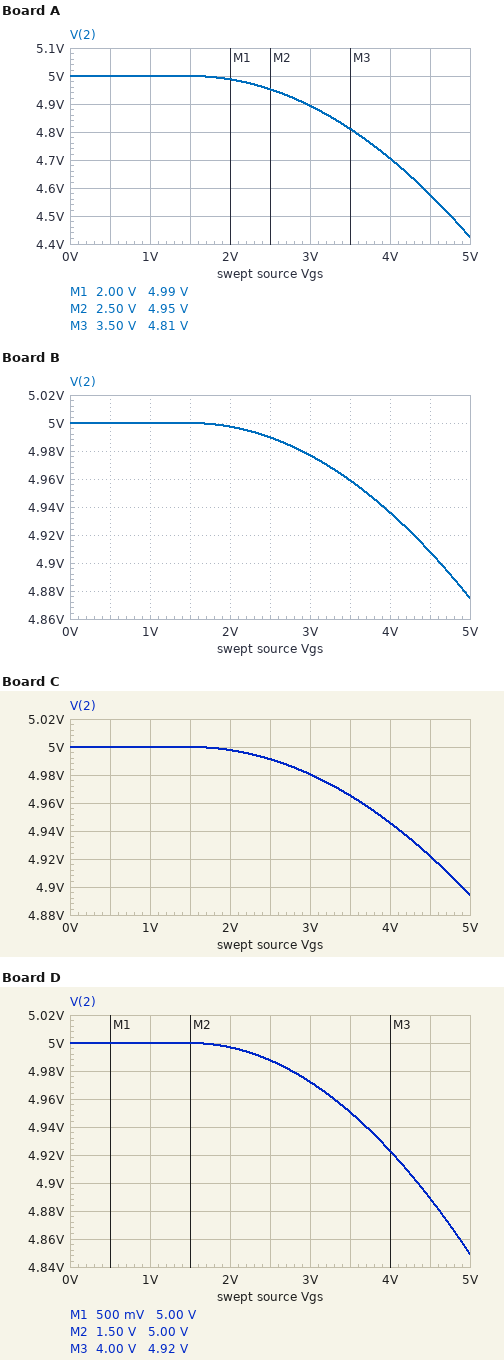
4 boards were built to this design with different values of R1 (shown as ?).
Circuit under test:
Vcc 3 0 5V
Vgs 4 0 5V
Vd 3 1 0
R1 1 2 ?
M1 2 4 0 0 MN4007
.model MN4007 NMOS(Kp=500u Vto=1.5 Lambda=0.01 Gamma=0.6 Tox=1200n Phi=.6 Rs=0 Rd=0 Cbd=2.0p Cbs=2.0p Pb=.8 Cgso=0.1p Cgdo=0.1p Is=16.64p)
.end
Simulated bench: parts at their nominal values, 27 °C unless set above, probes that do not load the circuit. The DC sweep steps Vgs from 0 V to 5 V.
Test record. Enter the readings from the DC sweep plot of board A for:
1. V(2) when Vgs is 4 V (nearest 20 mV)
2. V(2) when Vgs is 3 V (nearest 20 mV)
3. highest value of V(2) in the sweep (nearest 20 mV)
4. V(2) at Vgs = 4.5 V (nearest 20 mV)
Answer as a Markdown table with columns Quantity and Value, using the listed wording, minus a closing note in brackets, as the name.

| Quantity | Value |
|---|---|
| V(2) when Vgs is 4 V | 4.70 V |
| V(2) when Vgs is 3 V | 4.90 V |
| highest value of V(2) in the sweep | 5.00 V |
| V(2) at Vgs = 4.5 V | 4.58 V |
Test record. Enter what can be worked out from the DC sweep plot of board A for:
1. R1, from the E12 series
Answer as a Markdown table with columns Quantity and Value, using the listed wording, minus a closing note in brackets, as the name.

| Quantity | Value |
|---|---|
| R1, from the E12 series | 180 Ω |
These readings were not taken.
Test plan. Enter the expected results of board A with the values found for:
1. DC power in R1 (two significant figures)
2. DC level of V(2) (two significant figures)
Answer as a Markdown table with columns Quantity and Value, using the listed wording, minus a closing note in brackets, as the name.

| Quantity | Value |
|---|---|
| DC power in R1 | 1.8 mW |
| DC level of V(2) | 4.4 V |
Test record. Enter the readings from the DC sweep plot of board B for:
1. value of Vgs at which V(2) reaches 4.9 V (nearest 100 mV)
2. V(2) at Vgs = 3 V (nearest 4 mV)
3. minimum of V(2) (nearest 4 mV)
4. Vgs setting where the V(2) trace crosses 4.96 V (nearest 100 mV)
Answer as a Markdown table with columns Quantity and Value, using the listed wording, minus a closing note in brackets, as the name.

| Quantity | Value |
|---|---|
| value of Vgs at which V(2) reaches 4.9 V | 4.6 V |
| V(2) at Vgs = 3 V | 4.976 V |
| minimum of V(2) | 4.876 V |
| Vgs setting where the V(2) trace crosses 4.96 V | 3.5 V |
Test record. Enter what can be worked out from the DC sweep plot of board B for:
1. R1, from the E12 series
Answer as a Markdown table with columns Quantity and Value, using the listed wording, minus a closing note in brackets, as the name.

| Quantity | Value |
|---|---|
| R1, from the E12 series | 39 Ω |
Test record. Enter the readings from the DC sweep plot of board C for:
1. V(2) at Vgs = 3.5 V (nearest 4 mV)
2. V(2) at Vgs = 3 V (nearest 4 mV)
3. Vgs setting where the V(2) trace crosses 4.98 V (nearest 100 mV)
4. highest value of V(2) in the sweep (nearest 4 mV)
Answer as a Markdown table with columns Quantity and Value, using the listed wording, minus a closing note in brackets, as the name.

| Quantity | Value |
|---|---|
| V(2) at Vgs = 3.5 V | 4.964 V |
| V(2) at Vgs = 3 V | 4.980 V |
| Vgs setting where the V(2) trace crosses 4.98 V | 3.0 V |
| highest value of V(2) in the sweep | 5.000 V |
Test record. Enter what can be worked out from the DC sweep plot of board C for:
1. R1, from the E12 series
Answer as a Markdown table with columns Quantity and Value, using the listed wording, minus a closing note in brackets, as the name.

| Quantity | Value |
|---|---|
| R1, from the E12 series | 33 Ω |
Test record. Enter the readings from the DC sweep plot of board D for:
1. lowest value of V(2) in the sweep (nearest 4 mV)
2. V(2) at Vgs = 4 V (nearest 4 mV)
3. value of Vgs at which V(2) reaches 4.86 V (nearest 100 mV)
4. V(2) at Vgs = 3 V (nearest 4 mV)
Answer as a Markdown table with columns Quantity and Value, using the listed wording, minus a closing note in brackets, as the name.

| Quantity | Value |
|---|---|
| lowest value of V(2) in the sweep | 4.848 V |
| V(2) at Vgs = 4 V | 4.924 V |
| value of Vgs at which V(2) reaches 4.86 V | 4.9 V |
| V(2) at Vgs = 3 V | 4.972 V |
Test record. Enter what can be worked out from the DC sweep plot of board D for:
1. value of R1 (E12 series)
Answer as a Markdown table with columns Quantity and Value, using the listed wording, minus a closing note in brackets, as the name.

| Quantity | Value |
|---|---|
| value of R1 | 47 Ω |
